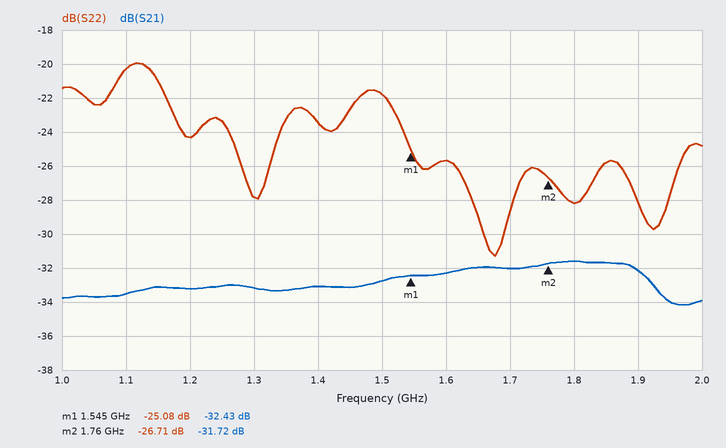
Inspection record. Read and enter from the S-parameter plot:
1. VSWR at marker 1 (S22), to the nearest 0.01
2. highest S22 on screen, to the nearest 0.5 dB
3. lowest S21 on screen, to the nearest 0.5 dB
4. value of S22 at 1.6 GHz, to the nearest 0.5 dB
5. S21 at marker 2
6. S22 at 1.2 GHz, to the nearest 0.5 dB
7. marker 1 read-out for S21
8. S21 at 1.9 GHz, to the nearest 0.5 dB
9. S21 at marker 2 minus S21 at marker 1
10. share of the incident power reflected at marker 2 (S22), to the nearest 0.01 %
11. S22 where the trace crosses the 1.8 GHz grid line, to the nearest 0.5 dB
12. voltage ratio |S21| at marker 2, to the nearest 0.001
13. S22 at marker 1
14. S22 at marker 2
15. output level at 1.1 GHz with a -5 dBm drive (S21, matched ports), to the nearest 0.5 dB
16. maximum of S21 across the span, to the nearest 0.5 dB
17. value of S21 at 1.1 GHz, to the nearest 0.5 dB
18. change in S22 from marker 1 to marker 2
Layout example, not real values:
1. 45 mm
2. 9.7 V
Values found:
1. 1.12
2. -20.0 dB
3. -34.0 dB
4. -25.5 dB
5. -31.72 dB
6. -24.5 dB
7. -32.43 dB
8. -32.0 dB
9. 0.71 dB
10. 0.21 %
11. -28.0 dB
12. 0.026
13. -25.08 dB
14. -26.71 dB
15. -38.5 dBm
16. -31.5 dB
17. -33.5 dB
18. -1.63 dB
